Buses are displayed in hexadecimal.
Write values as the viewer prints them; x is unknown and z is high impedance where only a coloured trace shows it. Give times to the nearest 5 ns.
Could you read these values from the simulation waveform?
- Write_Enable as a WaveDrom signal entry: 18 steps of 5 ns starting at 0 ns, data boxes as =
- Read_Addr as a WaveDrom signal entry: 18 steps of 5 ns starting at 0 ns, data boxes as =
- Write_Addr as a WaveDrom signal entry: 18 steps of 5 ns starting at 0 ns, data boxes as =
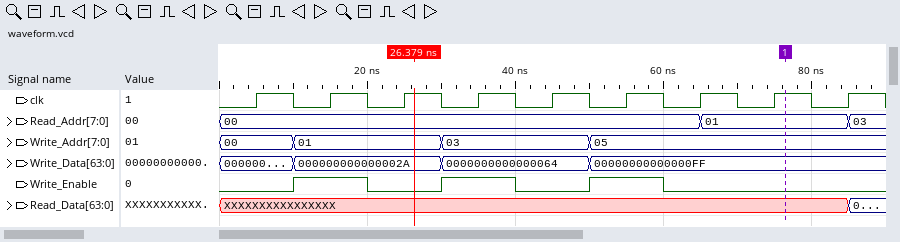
{name: 'Write_Enable', wave: '0.1.0.1.0.1.0.....'}
{name: 'Read_Addr', wave: '=............=...=', data: '00 01 03'}
{name: 'Write_Addr', wave: '=.=...=...=.......', data: '00 01 03 05'}
